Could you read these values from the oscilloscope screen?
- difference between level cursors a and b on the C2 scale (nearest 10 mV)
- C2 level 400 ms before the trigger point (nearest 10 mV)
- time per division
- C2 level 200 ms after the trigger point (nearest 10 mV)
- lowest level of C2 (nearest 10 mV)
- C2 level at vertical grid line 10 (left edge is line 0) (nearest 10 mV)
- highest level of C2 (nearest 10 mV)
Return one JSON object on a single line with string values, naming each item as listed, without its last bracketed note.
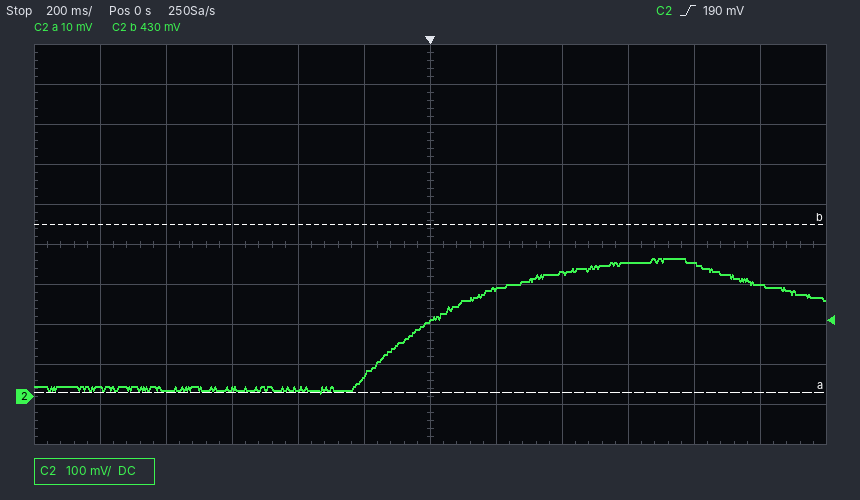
{"difference between level cursors a and b on the C2 scale": "420 mV", "C2 level 400 ms before the trigger point": "20 mV", "time per division": "200 ms", "C2 level 200 ms after the trigger point": "270 mV", "lowest level of C2": "10 mV", "C2 level at vertical grid line 10 (left edge is line 0)": "330 mV", "highest level of C2": "340 mV"}
